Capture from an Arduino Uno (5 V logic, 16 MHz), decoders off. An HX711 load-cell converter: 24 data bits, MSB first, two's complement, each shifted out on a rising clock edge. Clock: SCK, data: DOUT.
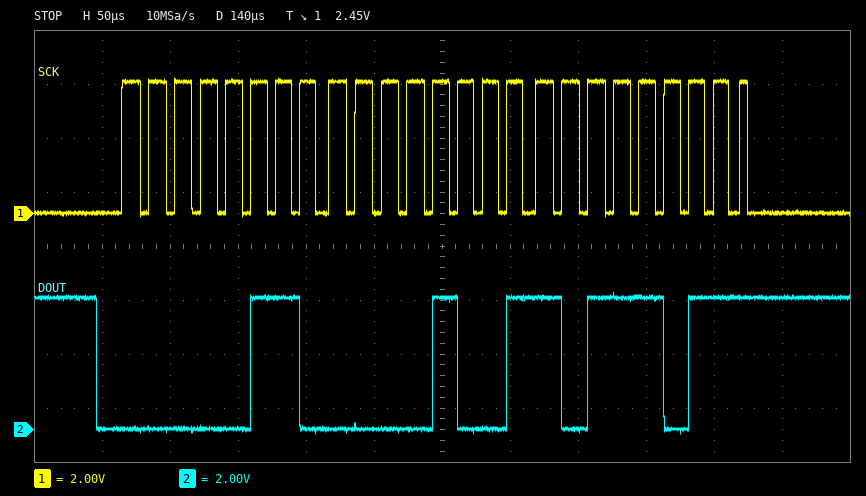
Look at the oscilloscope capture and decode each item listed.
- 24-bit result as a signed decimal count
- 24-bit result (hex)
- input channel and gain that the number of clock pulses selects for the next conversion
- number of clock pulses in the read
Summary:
395707
0x0609BB
channel A, gain 128
25
